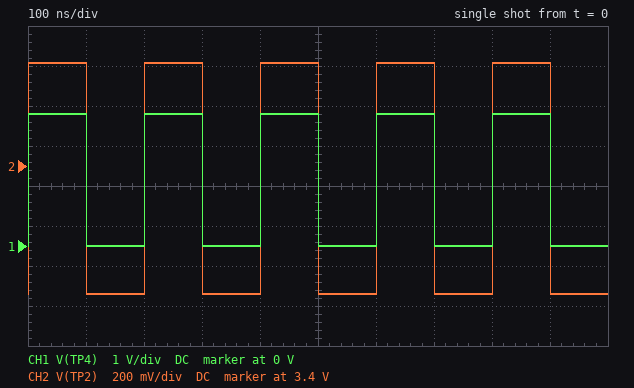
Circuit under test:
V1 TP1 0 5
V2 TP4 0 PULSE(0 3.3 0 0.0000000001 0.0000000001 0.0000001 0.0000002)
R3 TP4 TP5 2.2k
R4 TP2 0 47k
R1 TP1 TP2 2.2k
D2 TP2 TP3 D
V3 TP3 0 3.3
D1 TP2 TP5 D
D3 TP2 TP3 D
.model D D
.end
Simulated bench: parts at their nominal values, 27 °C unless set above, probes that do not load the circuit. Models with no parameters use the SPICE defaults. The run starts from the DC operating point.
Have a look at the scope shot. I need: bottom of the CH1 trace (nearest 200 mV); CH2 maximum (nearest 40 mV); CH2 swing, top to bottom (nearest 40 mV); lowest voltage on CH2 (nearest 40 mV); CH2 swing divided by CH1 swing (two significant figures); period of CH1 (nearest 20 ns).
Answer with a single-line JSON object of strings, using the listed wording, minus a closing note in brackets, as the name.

{"bottom of the CH1 trace": "0 V", "CH2 maximum": "3.92 V", "CH2 swing, top to bottom": "1.16 V", "lowest voltage on CH2": "2.76 V", "CH2 swing divided by CH1 swing": "0.35", "period of CH1": "200 ns"}
